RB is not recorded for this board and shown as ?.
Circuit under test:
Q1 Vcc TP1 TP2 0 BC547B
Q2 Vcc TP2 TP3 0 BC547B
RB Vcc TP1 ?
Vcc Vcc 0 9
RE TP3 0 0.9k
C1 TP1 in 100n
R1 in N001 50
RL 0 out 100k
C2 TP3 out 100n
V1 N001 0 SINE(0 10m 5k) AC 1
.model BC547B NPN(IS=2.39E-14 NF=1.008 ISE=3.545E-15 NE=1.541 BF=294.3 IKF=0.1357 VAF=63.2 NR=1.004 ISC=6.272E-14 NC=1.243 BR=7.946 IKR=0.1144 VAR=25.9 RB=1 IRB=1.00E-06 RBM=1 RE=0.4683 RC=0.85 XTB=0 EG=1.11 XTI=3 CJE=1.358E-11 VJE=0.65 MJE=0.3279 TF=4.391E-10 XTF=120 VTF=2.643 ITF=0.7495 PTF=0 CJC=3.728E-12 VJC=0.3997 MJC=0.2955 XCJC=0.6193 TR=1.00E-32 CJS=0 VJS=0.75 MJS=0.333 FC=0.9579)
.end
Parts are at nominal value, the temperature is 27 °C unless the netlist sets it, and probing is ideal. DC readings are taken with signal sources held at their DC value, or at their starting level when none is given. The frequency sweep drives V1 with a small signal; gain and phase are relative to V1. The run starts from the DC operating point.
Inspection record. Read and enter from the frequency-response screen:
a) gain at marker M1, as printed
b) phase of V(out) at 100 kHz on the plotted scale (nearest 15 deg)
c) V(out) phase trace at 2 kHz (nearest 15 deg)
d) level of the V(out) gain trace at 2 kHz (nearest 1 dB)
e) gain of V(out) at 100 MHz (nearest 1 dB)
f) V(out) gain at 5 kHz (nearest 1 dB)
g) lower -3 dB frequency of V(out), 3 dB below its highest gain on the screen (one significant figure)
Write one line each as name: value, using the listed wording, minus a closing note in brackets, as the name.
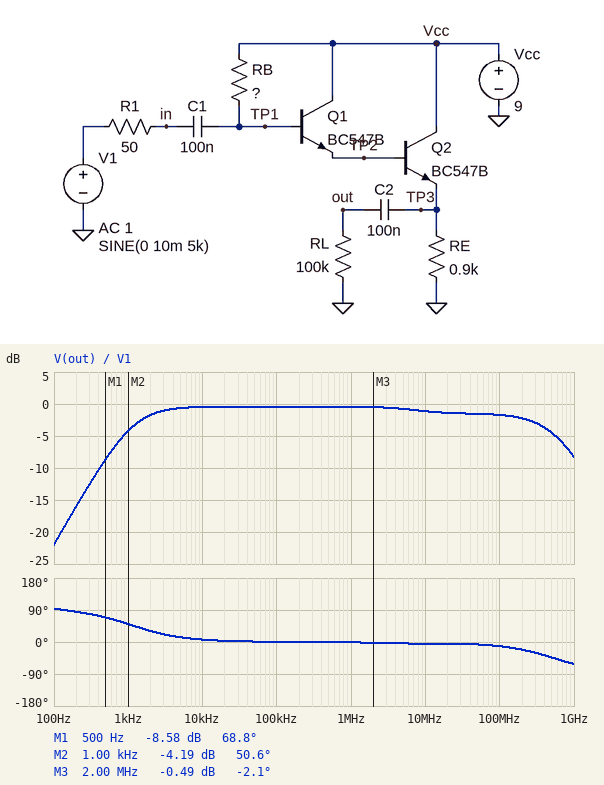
gain at marker M1, as printed: -8.58 dB
phase of V(out) at 100 kHz on the plotted scale: 0 deg
V(out) phase trace at 2 kHz: 30 deg
level of the V(out) gain trace at 2 kHz: -2 dB
gain of V(out) at 100 MHz: -2 dB
V(out) gain at 5 kHz: -1 dB
lower -3 dB frequency of V(out), 3 dB below its highest gain on the screen: 1 kHz
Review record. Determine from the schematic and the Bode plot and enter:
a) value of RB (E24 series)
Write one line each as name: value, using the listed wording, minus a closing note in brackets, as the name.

value of RB: 1.3 kΩ
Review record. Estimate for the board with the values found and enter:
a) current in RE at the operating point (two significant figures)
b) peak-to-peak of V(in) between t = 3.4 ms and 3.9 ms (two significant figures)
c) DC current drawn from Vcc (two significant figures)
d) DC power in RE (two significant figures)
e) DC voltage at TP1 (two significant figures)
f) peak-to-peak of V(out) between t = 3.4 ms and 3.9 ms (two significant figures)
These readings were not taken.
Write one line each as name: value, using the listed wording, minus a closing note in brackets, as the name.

current in RE at the operating point: 8.6 mA
peak-to-peak of V(in) between t = 3.4 ms and 3.9 ms: 19 mV
DC current drawn from Vcc: 8.6 mA
DC power in RE: 67 mW
DC voltage at TP1: 9.0 V
peak-to-peak of V(out) between t = 3.4 ms and 3.9 ms: 19 mV
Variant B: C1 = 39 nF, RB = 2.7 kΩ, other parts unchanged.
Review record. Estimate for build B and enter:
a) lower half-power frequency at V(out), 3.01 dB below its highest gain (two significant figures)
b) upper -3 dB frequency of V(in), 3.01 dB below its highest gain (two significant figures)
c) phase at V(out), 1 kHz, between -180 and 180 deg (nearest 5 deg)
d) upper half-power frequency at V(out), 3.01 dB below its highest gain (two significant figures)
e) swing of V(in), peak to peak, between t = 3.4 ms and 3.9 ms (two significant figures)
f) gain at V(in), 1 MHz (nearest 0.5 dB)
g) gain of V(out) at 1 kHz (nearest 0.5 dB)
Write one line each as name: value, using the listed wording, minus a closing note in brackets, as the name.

lower half-power frequency at V(out), 3.01 dB below its highest gain: 1.5 kHz
upper -3 dB frequency of V(in), 3.01 dB below its highest gain: 460 MHz
phase at V(out), 1 kHz, between -180 and 180 deg: 55 deg
upper half-power frequency at V(out), 3.01 dB below its highest gain: 360 MHz
swing of V(in), peak to peak, between t = 3.4 ms and 3.9 ms: 20 mV
gain at V(in), 1 MHz: 0 dB
gain of V(out) at 1 kHz: -5.5 dB
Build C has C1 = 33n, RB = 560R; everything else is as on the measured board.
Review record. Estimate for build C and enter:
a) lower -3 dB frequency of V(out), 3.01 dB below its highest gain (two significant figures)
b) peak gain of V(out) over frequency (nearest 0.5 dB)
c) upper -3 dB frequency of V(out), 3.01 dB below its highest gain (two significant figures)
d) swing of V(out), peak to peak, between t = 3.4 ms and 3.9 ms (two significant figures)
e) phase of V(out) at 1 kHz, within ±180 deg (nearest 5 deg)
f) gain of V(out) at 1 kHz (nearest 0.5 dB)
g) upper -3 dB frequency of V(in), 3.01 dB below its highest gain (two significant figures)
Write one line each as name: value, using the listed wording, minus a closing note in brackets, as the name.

lower -3 dB frequency of V(out), 3.01 dB below its highest gain: 7.9 kHz
peak gain of V(out) over frequency: -1.0 dB
upper -3 dB frequency of V(out), 3.01 dB below its highest gain: 390 MHz
swing of V(out), peak to peak, between t = 3.4 ms and 3.9 ms: 9.7 mV
phase of V(out) at 1 kHz, within ±180 deg: 85 deg
gain of V(out) at 1 kHz: -19.0 dB
upper -3 dB frequency of V(in), 3.01 dB below its highest gain: 410 MHz
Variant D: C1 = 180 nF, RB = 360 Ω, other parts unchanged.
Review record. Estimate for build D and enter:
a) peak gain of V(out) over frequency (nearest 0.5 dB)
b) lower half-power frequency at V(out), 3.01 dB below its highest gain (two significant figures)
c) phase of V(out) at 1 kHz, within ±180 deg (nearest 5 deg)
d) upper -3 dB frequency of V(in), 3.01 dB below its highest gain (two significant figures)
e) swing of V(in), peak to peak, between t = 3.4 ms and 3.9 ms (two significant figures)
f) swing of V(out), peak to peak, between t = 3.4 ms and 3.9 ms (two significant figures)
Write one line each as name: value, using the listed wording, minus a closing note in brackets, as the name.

peak gain of V(out) over frequency: -1.0 dB
lower half-power frequency at V(out), 3.01 dB below its highest gain: 2.2 kHz
phase of V(out) at 1 kHz, within ±180 deg: 65 deg
upper -3 dB frequency of V(in), 3.01 dB below its highest gain: 380 MHz
swing of V(in), peak to peak, between t = 3.4 ms and 3.9 ms: 18 mV
swing of V(out), peak to peak, between t = 3.4 ms and 3.9 ms: 16 mV
